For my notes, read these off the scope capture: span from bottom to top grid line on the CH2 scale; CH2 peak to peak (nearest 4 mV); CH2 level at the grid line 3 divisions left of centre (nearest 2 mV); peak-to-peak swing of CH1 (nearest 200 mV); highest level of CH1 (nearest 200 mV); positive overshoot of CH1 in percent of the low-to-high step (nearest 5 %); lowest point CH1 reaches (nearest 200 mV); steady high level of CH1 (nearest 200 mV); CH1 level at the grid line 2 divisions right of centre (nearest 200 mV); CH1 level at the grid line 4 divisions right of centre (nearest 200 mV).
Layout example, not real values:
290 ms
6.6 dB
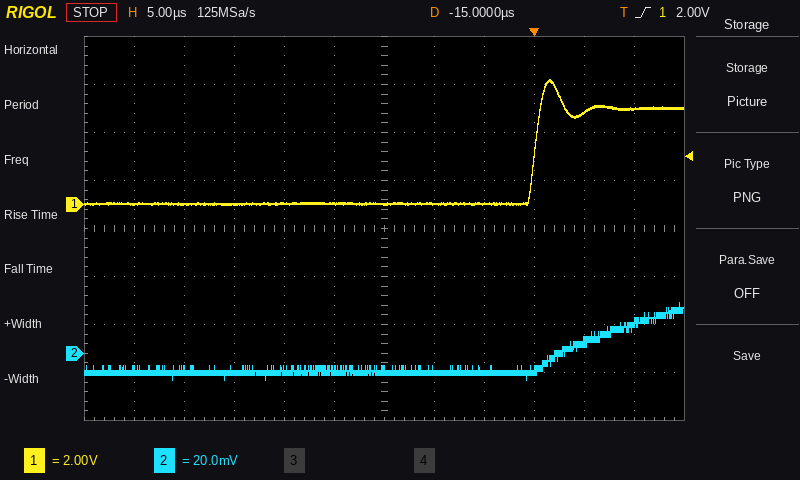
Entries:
160 mV
32 mV
-8 mV
5.2 V
5.2 V
30 %
0.0 V
4.0 V
0.0 V
3.8 V
